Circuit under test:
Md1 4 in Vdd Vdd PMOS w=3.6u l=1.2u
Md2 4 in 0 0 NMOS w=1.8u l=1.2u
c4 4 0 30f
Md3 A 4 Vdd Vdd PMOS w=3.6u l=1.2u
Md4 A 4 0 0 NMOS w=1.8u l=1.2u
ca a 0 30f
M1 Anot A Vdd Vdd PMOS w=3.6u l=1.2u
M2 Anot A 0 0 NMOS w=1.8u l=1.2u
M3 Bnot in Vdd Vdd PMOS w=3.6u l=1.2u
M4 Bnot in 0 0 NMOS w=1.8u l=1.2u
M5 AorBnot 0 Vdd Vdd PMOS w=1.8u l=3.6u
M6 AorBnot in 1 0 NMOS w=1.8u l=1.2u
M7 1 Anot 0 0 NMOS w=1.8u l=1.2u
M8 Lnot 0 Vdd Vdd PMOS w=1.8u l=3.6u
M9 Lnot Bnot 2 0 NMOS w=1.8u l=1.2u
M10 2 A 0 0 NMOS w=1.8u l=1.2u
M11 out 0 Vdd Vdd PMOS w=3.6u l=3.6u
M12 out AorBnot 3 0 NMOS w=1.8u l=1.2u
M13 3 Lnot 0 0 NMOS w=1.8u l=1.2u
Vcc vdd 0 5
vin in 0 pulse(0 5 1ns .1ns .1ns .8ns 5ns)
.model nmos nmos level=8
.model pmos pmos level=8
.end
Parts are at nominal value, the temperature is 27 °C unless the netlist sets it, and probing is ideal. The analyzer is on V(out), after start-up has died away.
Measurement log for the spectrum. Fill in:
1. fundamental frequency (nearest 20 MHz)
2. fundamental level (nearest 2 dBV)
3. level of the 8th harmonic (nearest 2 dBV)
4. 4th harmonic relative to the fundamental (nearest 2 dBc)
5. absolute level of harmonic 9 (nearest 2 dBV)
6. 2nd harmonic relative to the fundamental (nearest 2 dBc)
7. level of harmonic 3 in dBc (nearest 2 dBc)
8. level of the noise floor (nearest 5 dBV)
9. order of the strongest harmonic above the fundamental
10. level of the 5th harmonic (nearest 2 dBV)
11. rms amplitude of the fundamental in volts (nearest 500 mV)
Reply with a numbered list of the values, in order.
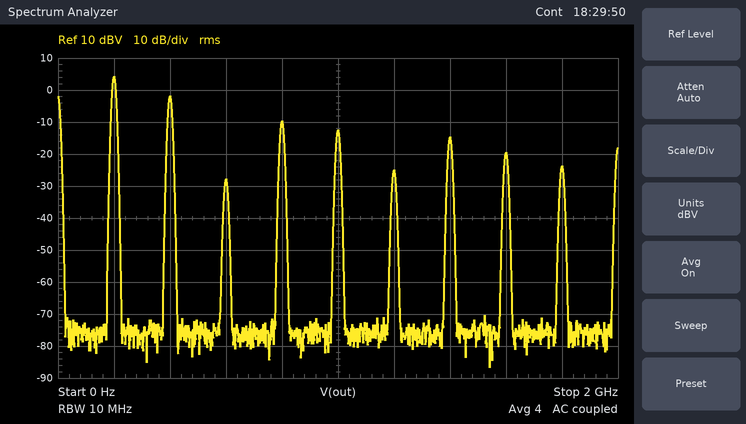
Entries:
1. 200 MHz
2. 4 dBV
3. -20 dBV
4. -14 dBc
5. -24 dBV
6. -6 dBc
7. -32 dBc
8. -75 dBV
9. 2
10. -12 dBV
11. 1.5 V
